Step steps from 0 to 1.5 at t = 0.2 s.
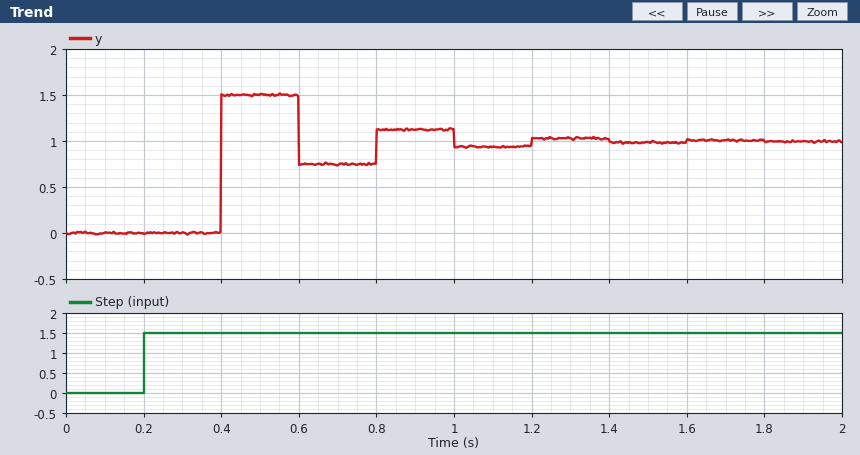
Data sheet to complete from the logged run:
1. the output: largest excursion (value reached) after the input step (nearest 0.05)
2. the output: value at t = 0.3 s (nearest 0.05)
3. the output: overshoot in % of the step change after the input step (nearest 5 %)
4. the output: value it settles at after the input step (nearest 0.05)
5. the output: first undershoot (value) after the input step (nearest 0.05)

1.50
0.00
50 %
1.00
0.75
